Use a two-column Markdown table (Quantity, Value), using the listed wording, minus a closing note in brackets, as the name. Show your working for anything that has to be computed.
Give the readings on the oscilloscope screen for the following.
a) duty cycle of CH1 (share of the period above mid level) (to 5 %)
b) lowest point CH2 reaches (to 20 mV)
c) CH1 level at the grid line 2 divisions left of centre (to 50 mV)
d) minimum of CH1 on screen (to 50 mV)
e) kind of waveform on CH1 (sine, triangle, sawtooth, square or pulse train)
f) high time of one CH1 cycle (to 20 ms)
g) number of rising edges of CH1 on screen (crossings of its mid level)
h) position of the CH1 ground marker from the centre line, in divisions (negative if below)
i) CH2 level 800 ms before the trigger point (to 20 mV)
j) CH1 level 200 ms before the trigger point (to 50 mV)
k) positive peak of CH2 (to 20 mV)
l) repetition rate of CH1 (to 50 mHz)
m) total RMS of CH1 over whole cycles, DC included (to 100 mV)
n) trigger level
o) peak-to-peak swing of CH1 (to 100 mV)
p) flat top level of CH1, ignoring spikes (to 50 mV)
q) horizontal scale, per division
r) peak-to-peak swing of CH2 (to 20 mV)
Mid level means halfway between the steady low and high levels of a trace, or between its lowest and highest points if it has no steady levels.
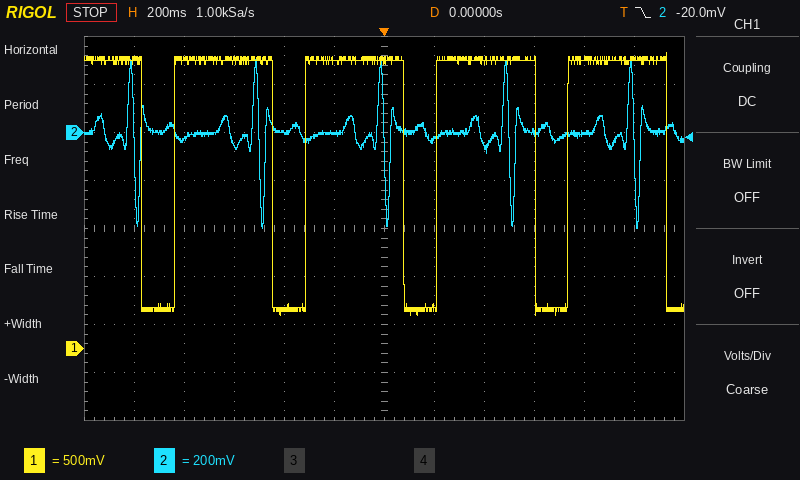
| Quantity | Value |
|---|---|
| duty cycle of CH1 (share of the period above mid level) | 75 % |
| lowest point CH2 reaches | -400 mV |
| CH1 level at the grid line 2 divisions left of centre | 400 mV |
| minimum of CH1 on screen | 350 mV |
| kind of waveform on CH1 | pulse train |
| high time of one CH1 cycle | 400 ms |
| number of rising edges of CH1 on screen | 4 |
| position of the CH1 ground marker from the centre line, in divisions | -2.5 div |
| CH2 level 800 ms before the trigger point | -20 mV |
| CH1 level 200 ms before the trigger point | 3.00 V |
| positive peak of CH2 | 300 mV |
| repetition rate of CH1 | 1.90 Hz |
| total RMS of CH1 over whole cycles, DC included | √(0.75 × (3.00 V)² + 0.25 × (350 mV)²) ≈ 2.6 V |
| trigger level | -20.0 mV |
| peak-to-peak swing of CH1 | 2.70 V |
| flat top level of CH1, ignoring spikes | 3.00 V |
| horizontal scale, per division | 200 ms |
| peak-to-peak swing of CH2 | 300 mV − (-400 mV) = 700 mV |
